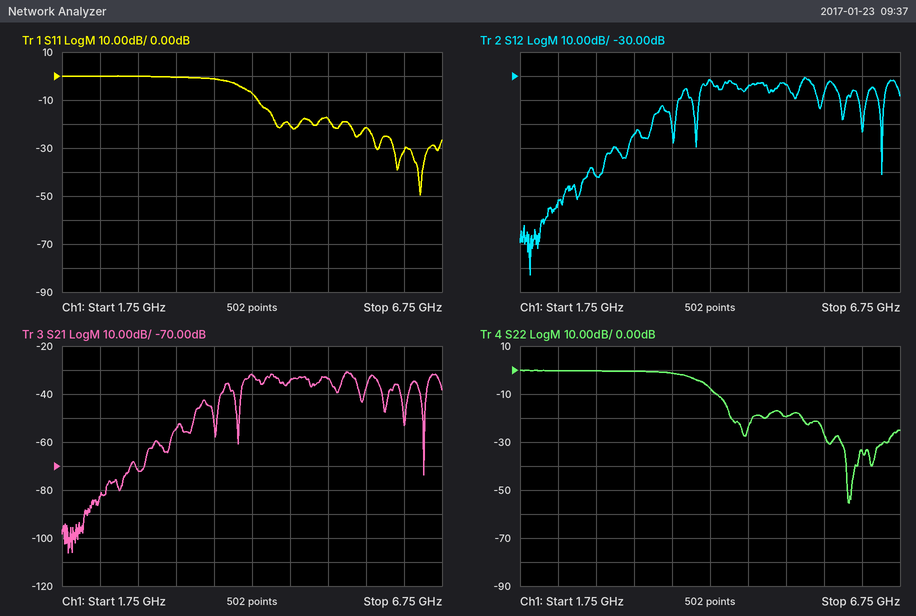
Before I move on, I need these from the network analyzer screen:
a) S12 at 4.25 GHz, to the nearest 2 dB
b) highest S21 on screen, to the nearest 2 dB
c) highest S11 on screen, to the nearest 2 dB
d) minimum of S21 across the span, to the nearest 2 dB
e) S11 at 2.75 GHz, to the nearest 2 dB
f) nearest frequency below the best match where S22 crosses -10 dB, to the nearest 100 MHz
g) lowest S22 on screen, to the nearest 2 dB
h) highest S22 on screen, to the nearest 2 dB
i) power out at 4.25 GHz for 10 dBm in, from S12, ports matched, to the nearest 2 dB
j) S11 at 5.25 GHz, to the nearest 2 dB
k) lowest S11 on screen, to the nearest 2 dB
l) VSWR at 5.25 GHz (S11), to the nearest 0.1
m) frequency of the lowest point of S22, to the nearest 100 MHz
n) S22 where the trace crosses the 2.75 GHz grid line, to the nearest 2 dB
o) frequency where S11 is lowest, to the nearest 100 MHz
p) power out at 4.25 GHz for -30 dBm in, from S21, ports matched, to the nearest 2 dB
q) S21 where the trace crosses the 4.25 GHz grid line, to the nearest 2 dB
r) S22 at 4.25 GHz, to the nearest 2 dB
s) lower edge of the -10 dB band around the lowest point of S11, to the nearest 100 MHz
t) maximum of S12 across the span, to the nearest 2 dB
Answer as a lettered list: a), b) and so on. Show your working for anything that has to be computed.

a) -32 dB
b) -30 dB
c) 0 dB
d) -106 dB
e) 0 dB
f) 4.3 GHz
g) -56 dB
h) 0 dB
i) 10 dBm + (-32 dB) = -22 dBm
j) -18 dB
k) -50 dB
l) |Γ| = 10^(-18/20) = 0.1259; VSWR = (1 + 0.1259)/(1 − 0.1259) ≈ 1.3
m) 6.1 GHz
n) 0 dB
o) 6.5 GHz
p) -30 dBm + (-32 dB) = -62 dBm
q) -32 dB
r) -8 dB
s) 4.3 GHz
t) -30 dB
